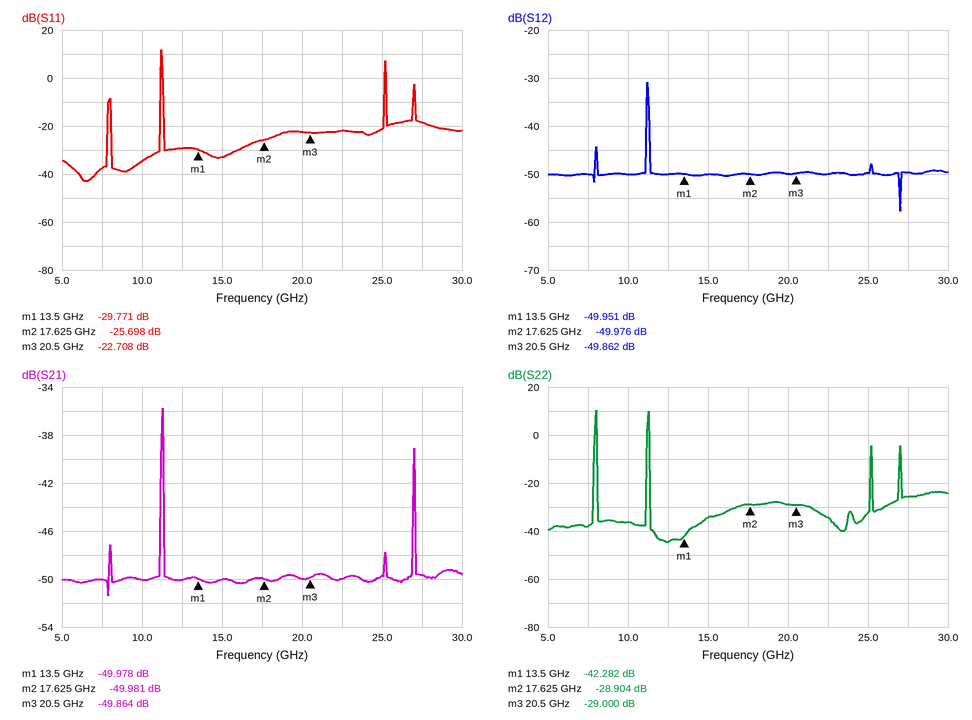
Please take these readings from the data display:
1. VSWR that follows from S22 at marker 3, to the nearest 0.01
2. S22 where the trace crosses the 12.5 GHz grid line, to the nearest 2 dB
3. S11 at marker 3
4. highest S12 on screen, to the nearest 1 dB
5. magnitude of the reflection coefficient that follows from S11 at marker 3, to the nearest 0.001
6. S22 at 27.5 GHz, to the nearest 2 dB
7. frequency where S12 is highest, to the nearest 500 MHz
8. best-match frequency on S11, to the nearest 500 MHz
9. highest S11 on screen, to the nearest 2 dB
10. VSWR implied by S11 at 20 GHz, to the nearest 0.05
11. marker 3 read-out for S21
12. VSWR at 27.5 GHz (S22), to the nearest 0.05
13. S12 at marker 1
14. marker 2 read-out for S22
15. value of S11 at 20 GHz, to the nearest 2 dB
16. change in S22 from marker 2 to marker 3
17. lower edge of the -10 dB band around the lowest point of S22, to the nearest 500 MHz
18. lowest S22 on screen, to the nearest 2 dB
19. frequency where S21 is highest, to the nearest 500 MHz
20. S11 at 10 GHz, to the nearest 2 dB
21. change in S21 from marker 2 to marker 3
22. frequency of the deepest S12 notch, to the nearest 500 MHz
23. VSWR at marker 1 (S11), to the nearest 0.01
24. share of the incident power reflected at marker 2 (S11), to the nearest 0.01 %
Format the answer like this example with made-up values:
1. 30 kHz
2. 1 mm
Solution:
1. 1.07
2. -44 dB
3. -22.708 dB
4. -31 dB
5. 0.073
6. -26 dB
7. 11.0 GHz
8. 6.5 GHz
9. 12 dB
10. 1.15
11. -49.864 dB
12. 1.10
13. -49.951 dB
14. -28.904 dB
15. -22 dB
16. -0.096 dB
17. 11.5 GHz
18. -44 dB
19. 11.5 GHz
20. -34 dB
21. 0.117 dB
22. 27.0 GHz
23. 1.07
24. 0.27 %
